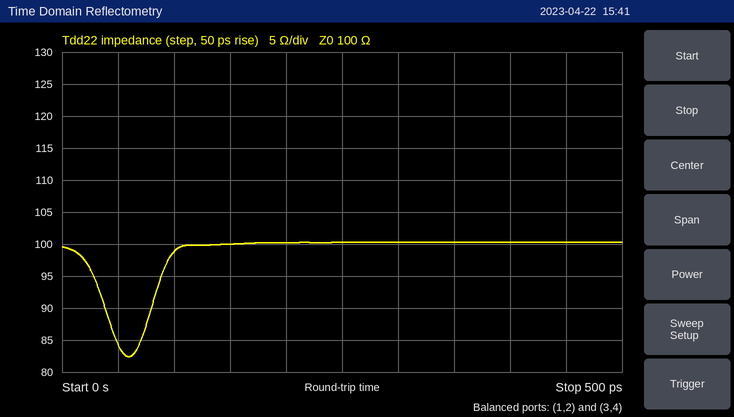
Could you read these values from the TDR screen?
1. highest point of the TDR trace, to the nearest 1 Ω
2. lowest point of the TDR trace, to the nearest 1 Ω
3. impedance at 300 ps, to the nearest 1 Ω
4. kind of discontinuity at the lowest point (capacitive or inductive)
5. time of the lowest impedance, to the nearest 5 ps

100 Ω
82 Ω
100 Ω
capacitive
60 ps
